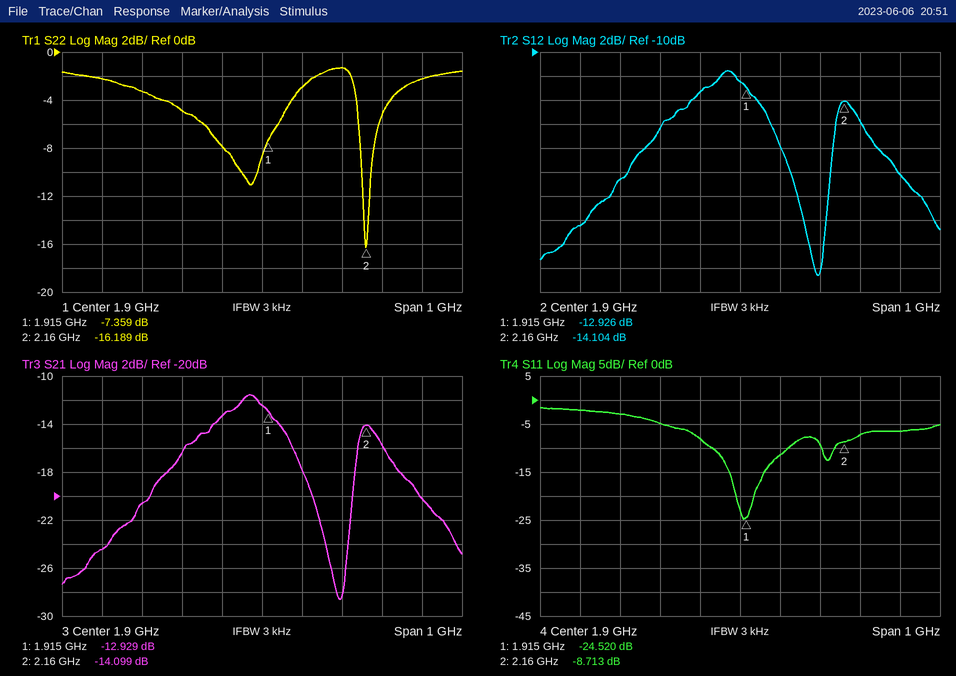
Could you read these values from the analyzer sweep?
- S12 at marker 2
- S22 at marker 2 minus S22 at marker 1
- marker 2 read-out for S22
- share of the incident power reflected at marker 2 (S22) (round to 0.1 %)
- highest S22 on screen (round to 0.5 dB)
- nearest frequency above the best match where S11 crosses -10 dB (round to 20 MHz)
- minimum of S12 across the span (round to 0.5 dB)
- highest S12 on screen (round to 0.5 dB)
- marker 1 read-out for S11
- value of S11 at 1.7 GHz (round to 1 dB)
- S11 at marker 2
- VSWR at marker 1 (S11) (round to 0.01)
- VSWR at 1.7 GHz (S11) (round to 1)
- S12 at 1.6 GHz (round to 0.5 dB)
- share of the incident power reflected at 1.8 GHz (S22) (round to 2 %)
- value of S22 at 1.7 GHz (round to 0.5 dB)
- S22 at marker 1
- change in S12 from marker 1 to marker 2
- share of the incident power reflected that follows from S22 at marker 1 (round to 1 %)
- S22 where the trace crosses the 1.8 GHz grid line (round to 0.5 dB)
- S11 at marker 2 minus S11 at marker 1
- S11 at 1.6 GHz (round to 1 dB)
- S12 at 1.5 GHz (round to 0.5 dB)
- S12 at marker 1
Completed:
-14.104 dB
-8.830 dB
-16.189 dB
2.4 %
-1.5 dB
2.02 GHz
-28.5 dB
-11.5 dB
-24.520 dB
-5 dB
-8.713 dB
1.13
4
-20.5 dB
16 %
-5.0 dB
-7.359 dB
-1.178 dB
18 %
-8.0 dB
15.807 dB
-3 dB
-24.5 dB
-12.926 dB
